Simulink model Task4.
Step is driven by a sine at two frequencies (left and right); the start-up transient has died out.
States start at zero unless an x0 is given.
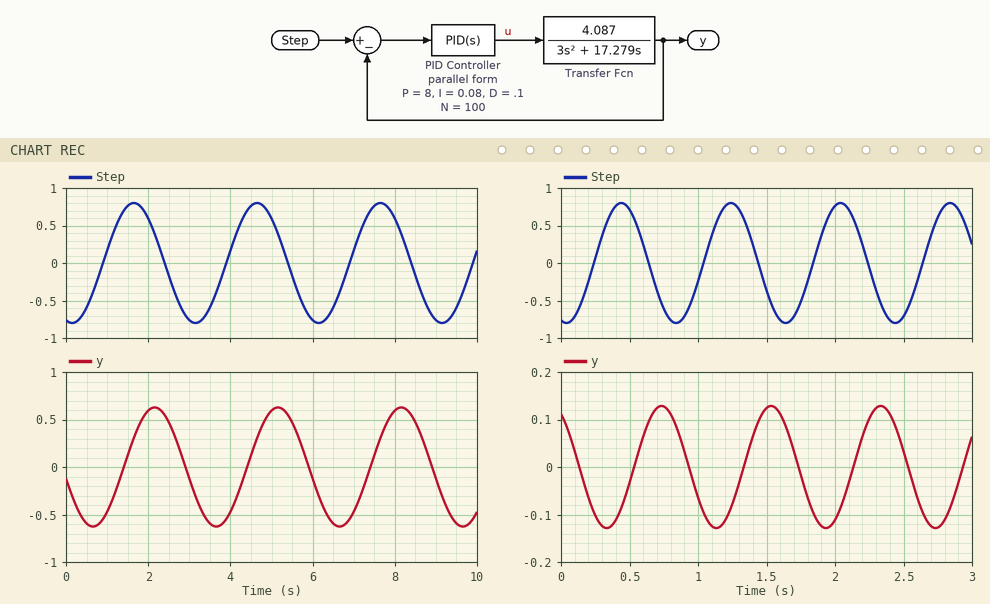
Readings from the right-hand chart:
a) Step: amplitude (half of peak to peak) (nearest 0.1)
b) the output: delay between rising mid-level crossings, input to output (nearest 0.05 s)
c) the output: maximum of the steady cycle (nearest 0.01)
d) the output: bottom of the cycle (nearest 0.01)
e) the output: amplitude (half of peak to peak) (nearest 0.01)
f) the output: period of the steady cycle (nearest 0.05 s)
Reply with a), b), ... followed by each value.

a) 0.8
b) 0.30 s
c) 0.13
d) -0.13
e) 0.13
f) 0.80 s
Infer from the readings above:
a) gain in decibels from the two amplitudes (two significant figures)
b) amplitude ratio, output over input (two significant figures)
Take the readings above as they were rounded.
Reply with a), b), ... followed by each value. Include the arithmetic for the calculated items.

a) 20 log10(0.13 / 0.8) = -16 dB
b) 0.13 / 0.8 = 0.16
